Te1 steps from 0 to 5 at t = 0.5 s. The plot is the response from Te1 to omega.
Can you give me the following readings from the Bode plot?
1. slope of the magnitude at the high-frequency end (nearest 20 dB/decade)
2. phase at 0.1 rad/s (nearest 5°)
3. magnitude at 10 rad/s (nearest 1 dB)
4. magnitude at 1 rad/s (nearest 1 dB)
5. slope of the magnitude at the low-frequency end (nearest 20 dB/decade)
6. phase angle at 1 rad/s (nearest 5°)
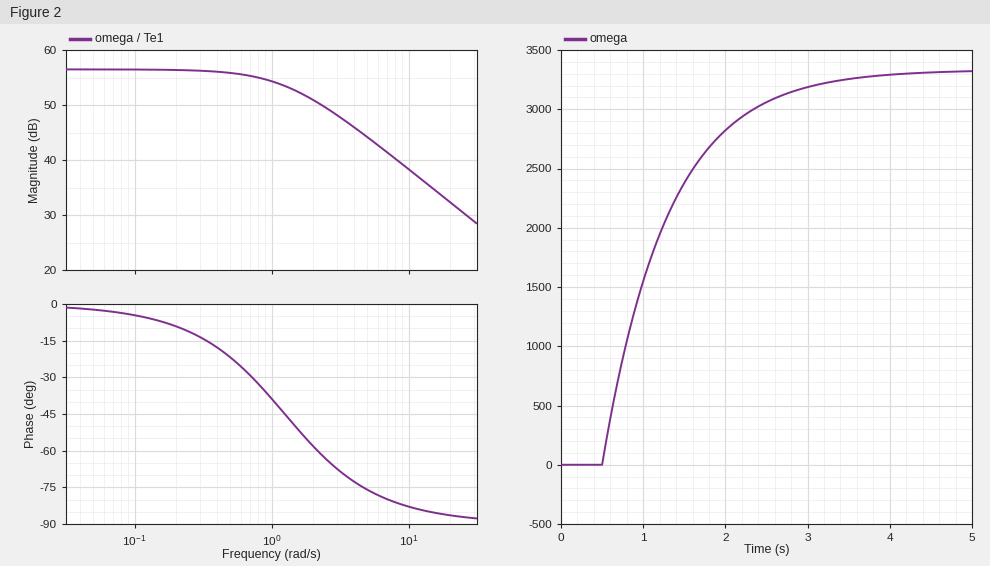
-20 dB/decade
-5°
38 dB
54 dB
0 dB/decade
-40°
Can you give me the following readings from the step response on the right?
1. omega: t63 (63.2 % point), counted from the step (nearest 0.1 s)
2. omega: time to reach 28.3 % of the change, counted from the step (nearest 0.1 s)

0.8 s
0.3 s
